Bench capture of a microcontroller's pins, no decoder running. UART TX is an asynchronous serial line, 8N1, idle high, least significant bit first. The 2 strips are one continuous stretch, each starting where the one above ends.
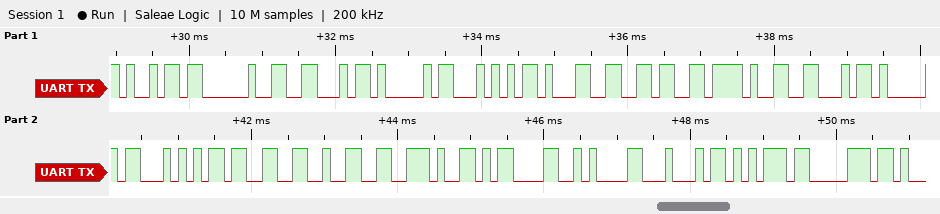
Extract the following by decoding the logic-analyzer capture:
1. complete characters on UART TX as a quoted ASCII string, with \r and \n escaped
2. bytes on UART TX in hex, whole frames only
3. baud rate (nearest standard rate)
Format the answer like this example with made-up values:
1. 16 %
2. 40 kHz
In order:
1. "i FAT16/FAT32.\r\nDup"
2. 0x69 0x20 0x46 0x41 0x54 0x31 0x36 0x2F 0x46 0x41 0x54 0x33 0x32 0x2E 0x0D 0x0A 0x44 0x75 0x70
3. 9600 baud
